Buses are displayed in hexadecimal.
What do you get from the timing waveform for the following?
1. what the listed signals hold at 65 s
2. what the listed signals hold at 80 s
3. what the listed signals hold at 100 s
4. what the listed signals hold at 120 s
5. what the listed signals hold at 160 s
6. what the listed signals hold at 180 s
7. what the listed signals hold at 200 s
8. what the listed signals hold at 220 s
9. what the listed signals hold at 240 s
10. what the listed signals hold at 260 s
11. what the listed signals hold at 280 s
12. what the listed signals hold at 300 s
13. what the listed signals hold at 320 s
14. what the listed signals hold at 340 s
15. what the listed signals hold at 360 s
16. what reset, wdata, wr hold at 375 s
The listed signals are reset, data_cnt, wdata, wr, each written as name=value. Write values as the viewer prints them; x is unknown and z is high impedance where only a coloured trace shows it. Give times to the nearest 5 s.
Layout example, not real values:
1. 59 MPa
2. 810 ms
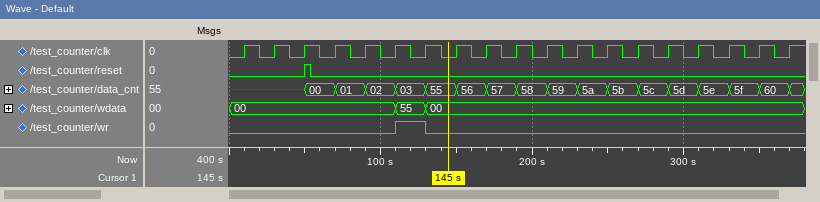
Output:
1. reset=0, data_cnt=00, wdata=00, wr=0
2. reset=0, data_cnt=01, wdata=00, wr=0
3. reset=0, data_cnt=02, wdata=00, wr=0
4. reset=0, data_cnt=03, wdata=55, wr=1
5. reset=0, data_cnt=56, wdata=00, wr=0
6. reset=0, data_cnt=57, wdata=00, wr=0
7. reset=0, data_cnt=58, wdata=00, wr=0
8. reset=0, data_cnt=59, wdata=00, wr=0
9. reset=0, data_cnt=5a, wdata=00, wr=0
10. reset=0, data_cnt=5b, wdata=00, wr=0
11. reset=0, data_cnt=5c, wdata=00, wr=0
12. reset=0, data_cnt=5d, wdata=00, wr=0
13. reset=0, data_cnt=5e, wdata=00, wr=0
14. reset=0, data_cnt=5f, wdata=00, wr=0
15. reset=0, data_cnt=60, wdata=00, wr=0
16. reset=0, wdata=00, wr=0
